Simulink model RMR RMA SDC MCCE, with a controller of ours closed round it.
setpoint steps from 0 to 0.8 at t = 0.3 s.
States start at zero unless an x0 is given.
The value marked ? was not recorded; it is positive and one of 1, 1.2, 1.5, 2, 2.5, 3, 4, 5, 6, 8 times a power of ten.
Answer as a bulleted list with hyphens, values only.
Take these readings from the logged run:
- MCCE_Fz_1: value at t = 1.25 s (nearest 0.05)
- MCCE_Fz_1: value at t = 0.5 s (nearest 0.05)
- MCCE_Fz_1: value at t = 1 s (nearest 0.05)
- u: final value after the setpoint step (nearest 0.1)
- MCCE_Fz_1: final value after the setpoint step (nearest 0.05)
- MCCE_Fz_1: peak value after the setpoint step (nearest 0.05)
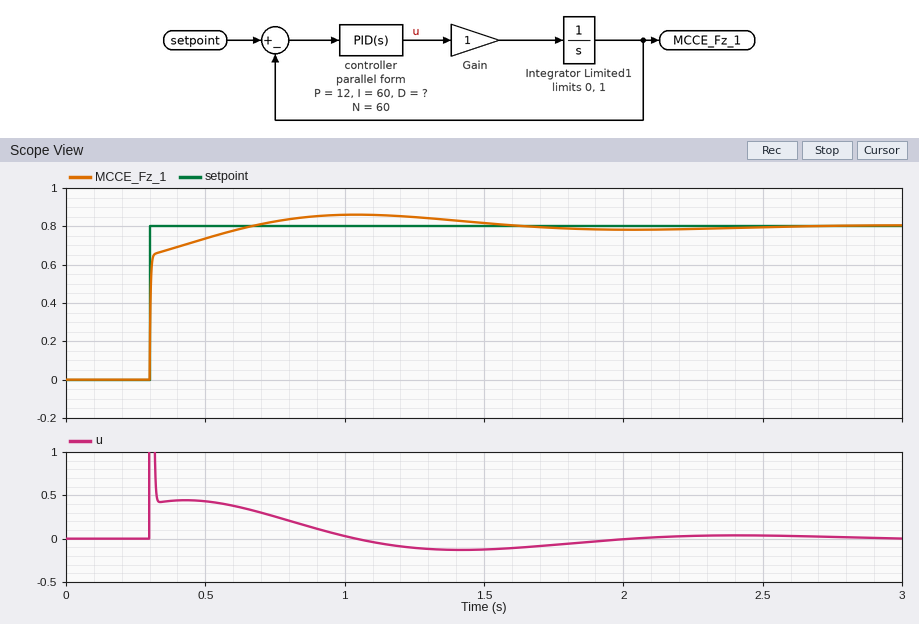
- 0.85
- 0.75
- 0.85
- 0.0
- 0.80
- 0.85
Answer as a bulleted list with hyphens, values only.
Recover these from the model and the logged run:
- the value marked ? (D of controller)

- 4
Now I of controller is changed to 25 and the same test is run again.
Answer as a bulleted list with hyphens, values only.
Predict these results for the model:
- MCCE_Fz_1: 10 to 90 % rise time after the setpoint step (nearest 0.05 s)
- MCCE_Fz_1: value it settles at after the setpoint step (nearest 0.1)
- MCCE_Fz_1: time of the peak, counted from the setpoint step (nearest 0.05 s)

- 0.20 s
- 0.8
- 1.05 s
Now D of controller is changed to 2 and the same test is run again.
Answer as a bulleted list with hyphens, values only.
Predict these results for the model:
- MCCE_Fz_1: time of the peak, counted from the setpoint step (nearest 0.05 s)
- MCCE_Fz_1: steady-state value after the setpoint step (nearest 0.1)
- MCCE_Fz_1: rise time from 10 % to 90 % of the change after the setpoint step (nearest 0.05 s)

- 0.55 s
- 0.8
- 0.15 s
